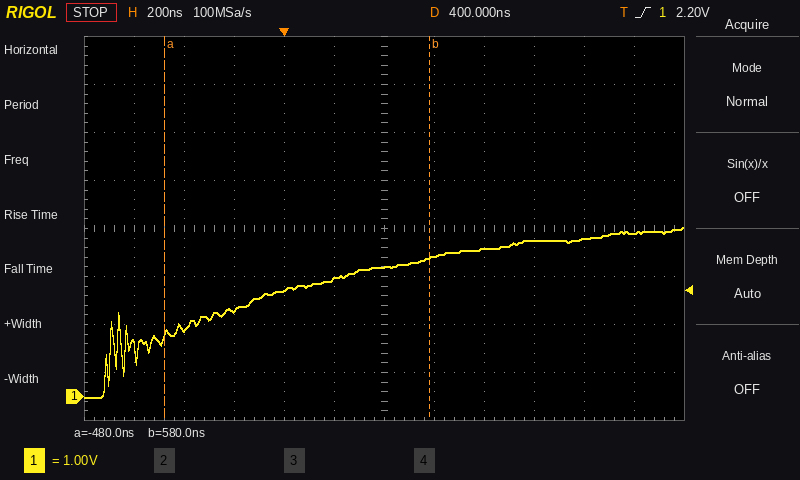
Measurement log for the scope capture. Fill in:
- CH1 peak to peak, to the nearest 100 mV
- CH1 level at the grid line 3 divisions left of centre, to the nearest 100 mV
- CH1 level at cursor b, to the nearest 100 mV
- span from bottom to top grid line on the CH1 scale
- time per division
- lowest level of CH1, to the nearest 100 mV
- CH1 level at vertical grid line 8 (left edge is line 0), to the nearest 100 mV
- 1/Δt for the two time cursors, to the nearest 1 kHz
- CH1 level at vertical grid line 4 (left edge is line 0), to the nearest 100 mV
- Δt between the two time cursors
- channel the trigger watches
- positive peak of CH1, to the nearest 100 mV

3.5 V
1.8 V
2.9 V
8 V
200 ns
0.0 V
3.1 V
943 kHz
2.2 V
1.06 µs
CH1
3.5 V
